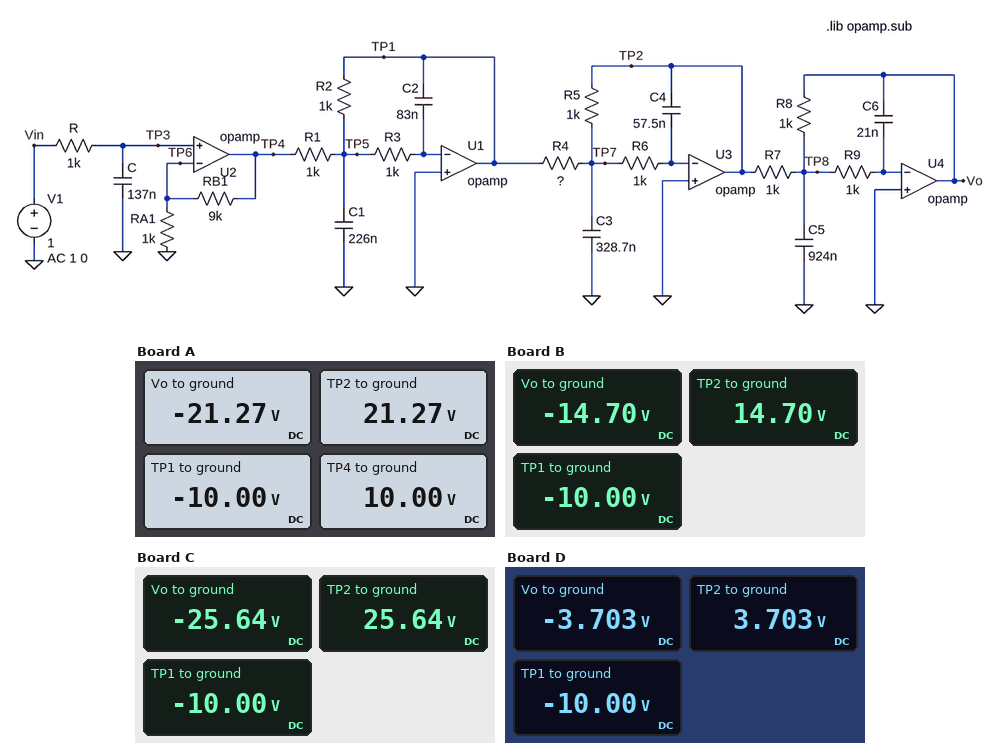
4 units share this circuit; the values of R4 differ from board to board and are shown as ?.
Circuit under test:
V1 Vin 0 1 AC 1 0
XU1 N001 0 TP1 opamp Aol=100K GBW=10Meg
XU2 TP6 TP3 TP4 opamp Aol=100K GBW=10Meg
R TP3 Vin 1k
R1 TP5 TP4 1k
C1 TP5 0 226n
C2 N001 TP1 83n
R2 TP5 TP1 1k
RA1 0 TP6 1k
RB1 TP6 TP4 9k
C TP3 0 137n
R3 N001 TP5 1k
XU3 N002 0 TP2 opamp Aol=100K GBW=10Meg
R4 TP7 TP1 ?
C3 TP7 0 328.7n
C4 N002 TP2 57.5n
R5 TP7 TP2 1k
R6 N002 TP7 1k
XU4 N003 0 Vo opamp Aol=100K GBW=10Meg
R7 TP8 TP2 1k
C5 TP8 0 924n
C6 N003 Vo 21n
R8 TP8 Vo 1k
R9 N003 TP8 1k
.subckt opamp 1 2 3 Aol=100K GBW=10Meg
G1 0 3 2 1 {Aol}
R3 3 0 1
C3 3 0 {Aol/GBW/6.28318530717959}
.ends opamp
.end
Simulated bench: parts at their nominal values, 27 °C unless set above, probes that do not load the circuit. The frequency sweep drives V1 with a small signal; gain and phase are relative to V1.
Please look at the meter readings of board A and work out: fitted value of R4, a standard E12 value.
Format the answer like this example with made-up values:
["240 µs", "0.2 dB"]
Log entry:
["470 Ω"]
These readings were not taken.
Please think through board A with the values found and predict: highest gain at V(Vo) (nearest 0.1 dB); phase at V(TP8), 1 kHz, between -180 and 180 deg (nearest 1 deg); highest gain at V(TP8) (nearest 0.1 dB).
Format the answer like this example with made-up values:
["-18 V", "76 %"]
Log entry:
["26.6 dB", "-171 deg", "5.7 dB"]
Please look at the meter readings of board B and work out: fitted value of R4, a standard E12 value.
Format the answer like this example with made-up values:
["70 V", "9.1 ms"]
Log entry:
["680 Ω"]
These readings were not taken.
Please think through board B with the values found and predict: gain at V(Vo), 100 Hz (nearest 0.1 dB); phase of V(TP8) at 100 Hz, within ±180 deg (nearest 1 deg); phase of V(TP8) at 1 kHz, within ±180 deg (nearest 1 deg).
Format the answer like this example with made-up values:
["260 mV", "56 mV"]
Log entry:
["23.3 dB", "67 deg", "-169 deg"]
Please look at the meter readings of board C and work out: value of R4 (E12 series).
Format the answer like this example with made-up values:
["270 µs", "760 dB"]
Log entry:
["390 Ω"]
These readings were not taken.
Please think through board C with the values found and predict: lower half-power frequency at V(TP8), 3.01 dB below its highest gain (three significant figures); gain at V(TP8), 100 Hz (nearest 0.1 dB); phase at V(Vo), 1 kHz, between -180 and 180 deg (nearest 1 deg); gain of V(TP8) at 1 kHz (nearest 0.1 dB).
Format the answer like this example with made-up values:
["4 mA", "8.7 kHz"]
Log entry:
["533 Hz", "-9.5 dB", "-82 deg", "6.5 dB"]
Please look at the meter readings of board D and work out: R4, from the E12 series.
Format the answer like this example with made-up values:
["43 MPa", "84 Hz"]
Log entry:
["2.7 kΩ"]
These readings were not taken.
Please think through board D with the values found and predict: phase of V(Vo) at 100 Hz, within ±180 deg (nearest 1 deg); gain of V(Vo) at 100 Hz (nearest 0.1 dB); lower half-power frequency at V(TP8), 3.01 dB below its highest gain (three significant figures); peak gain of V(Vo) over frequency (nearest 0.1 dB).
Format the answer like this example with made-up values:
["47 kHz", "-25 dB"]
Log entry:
["159 deg", "11.4 dB", "722 Hz", "12.9 dB"]
